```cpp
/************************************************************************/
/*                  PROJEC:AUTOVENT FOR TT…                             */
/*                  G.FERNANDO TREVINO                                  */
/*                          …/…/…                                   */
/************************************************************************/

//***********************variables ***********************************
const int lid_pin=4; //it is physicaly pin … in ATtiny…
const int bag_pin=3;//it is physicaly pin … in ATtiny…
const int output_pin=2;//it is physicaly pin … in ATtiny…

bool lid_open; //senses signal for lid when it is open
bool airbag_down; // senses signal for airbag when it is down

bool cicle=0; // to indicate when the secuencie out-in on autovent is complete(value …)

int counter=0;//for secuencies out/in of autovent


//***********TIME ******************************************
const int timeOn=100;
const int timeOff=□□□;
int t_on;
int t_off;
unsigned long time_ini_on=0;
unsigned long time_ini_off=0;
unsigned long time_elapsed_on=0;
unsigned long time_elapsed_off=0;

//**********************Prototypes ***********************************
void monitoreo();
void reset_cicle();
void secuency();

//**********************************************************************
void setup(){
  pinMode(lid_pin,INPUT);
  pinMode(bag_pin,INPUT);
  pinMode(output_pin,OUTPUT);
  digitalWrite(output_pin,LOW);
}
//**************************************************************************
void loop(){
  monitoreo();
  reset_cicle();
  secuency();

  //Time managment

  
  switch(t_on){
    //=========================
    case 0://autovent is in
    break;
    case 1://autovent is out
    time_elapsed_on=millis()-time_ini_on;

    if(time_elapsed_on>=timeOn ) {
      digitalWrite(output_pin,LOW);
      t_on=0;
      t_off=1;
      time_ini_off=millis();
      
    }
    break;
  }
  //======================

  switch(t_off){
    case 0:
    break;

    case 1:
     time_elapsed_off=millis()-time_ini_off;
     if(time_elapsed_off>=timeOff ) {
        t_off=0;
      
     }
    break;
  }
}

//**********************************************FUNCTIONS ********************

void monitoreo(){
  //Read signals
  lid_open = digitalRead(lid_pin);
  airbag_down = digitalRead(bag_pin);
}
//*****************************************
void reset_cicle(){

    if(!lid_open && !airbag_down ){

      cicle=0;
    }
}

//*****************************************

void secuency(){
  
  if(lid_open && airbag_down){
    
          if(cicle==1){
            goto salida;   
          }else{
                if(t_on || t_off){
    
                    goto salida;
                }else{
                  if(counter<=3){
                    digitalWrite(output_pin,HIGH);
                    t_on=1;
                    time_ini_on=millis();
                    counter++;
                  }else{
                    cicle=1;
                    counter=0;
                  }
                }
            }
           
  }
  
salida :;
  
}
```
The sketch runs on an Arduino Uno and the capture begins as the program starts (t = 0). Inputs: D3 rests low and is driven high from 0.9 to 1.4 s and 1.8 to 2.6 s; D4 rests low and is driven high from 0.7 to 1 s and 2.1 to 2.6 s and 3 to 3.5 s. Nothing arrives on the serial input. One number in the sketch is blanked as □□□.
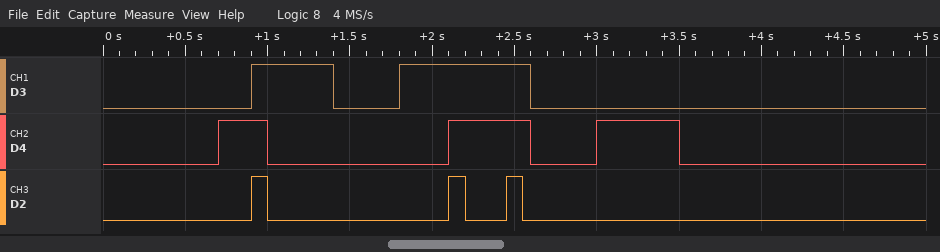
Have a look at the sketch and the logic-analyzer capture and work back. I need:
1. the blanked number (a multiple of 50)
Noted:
250
